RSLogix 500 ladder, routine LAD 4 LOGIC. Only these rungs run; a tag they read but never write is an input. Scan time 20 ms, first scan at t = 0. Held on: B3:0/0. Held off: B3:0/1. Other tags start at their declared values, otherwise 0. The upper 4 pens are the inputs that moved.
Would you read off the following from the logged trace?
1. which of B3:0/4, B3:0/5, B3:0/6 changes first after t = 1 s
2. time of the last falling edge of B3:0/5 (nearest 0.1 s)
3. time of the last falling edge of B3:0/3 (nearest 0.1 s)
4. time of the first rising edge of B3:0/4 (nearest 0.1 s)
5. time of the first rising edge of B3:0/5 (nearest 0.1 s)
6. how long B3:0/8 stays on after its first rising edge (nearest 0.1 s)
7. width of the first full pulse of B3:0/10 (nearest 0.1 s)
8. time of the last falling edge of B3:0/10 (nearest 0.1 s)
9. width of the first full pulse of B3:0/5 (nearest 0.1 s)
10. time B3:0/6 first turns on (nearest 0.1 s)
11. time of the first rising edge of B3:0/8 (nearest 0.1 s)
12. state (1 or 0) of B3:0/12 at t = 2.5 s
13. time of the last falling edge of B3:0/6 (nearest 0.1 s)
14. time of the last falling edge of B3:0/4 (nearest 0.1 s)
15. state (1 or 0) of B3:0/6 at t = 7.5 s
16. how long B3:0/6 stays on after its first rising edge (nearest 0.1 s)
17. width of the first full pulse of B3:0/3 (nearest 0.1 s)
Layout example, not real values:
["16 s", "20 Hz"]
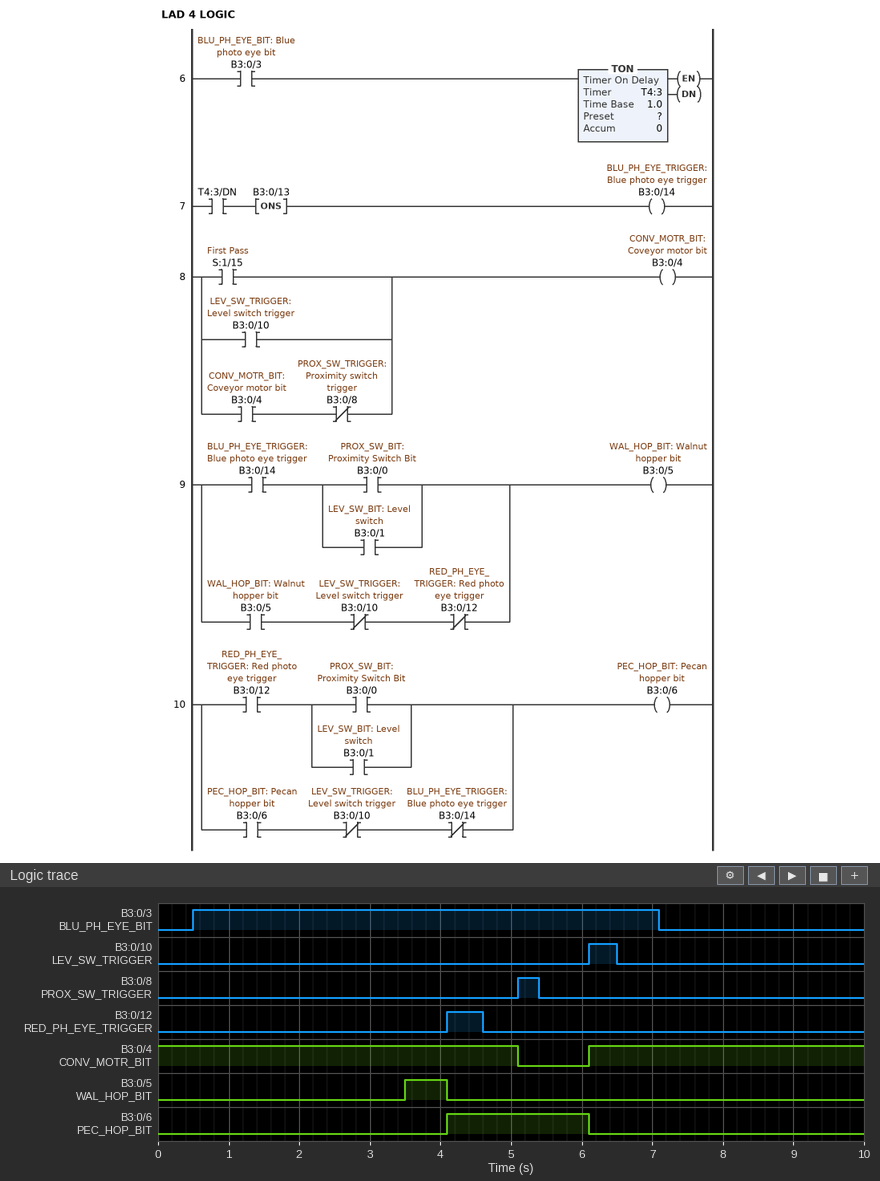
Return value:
["B3:0/5", "4.1 s", "7.1 s", "6.1 s", "3.5 s", "0.3 s", "0.4 s", "6.5 s", "0.6 s", "4.1 s", "5.1 s", "0", "6.1 s", "5.1 s", "0", "2.0 s", "6.6 s"]
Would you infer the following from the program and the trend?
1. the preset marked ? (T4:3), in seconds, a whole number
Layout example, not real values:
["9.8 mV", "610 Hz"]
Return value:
["3 s"]
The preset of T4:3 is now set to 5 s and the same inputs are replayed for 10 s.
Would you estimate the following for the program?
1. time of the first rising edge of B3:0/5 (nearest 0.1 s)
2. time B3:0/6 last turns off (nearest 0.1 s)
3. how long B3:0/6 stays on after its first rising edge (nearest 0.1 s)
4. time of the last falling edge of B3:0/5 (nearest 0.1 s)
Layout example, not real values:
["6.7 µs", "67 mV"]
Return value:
["5.5 s", "5.5 s", "1.4 s", "6.1 s"]
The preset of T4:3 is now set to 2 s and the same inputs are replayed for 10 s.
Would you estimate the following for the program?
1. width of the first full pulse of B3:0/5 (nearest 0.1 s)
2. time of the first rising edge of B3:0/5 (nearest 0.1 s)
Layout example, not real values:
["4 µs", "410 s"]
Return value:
["1.6 s", "2.5 s"]
